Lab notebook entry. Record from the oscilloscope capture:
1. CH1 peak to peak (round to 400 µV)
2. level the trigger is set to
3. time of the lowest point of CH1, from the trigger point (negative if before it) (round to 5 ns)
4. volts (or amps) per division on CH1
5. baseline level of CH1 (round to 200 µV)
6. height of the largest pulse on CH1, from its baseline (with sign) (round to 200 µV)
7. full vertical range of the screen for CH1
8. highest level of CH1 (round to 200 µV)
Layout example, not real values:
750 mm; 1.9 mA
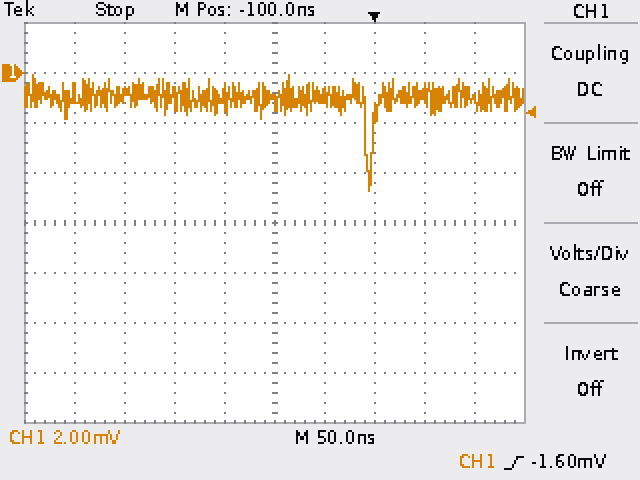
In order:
4.8 mV; -1.60 mV; -5 ns; 2 mV; -1.0 mV; -3.8 mV; 16 mV; 0.0 mV
